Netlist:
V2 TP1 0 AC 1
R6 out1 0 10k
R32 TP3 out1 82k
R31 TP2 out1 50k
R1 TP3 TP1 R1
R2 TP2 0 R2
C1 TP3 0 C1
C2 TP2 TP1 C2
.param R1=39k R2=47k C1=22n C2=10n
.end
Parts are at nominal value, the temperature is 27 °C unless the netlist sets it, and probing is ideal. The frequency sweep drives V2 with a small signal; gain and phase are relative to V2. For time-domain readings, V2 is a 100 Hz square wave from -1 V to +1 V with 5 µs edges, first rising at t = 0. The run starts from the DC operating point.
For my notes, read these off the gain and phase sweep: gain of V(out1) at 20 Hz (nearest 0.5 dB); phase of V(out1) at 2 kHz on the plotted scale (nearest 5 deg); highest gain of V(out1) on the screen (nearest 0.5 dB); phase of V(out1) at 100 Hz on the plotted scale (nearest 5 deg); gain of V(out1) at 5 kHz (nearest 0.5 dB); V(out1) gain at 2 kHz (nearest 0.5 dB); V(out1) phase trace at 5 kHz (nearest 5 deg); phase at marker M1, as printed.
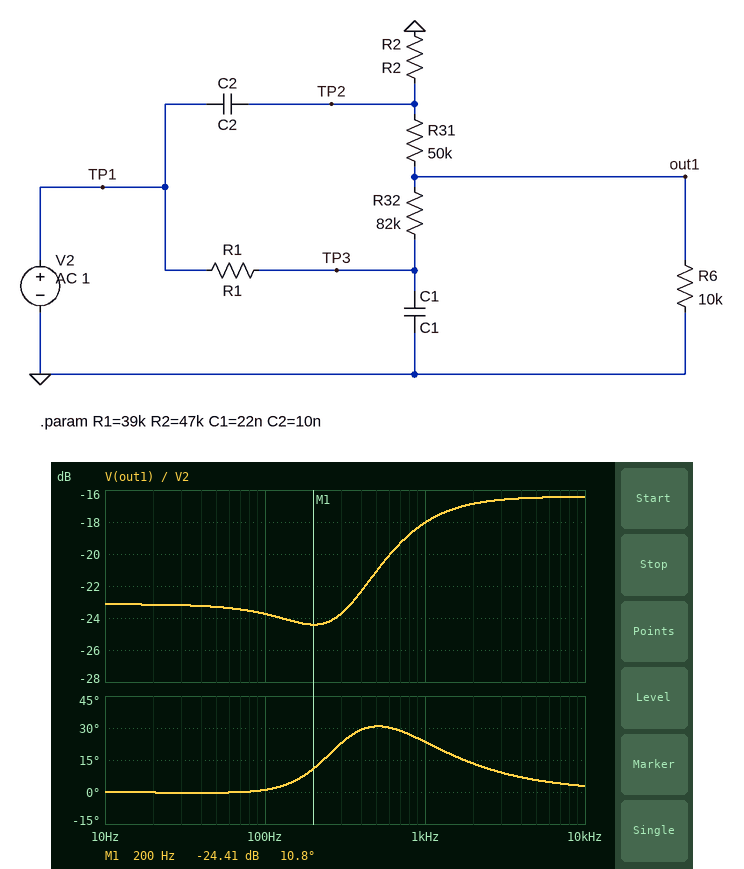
-23.0 dB
15 deg
-16.5 dB
0 deg
-16.5 dB
-17.0 dB
5 deg
10.8 deg
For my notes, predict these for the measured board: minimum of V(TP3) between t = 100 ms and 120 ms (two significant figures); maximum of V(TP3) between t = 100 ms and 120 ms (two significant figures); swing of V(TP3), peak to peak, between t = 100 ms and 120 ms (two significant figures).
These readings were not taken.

-700 mV
700 mV
1.4 V
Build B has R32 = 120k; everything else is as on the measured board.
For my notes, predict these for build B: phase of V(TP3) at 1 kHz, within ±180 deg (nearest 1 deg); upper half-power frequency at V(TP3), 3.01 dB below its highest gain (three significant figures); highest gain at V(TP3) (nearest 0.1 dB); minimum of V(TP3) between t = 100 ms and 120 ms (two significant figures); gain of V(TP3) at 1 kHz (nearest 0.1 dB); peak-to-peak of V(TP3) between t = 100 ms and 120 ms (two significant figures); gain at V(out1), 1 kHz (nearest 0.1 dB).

-75 deg
245 Hz
-2.3 dB
-770 mV
-14.6 dB
1.5 V
-17.7 dB
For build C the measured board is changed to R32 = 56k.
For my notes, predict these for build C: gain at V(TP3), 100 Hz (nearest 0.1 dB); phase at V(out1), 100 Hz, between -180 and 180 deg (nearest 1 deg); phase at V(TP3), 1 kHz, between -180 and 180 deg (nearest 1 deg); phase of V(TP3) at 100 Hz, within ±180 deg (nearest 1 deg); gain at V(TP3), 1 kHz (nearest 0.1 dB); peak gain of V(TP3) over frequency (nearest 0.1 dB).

-4.5 dB
-2 deg
-71 deg
-18 deg
-14.4 dB
-4.1 dB
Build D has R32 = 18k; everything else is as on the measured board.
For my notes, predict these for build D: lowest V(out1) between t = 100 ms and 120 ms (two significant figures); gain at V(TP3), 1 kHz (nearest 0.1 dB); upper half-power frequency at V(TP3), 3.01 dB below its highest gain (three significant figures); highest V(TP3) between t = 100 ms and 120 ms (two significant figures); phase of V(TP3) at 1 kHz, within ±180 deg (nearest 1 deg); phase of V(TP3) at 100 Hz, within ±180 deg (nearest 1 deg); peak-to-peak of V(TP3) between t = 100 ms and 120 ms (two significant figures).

-140 mV
-14.0 dB
545 Hz
410 mV
-60 deg
-10 deg
820 mV
